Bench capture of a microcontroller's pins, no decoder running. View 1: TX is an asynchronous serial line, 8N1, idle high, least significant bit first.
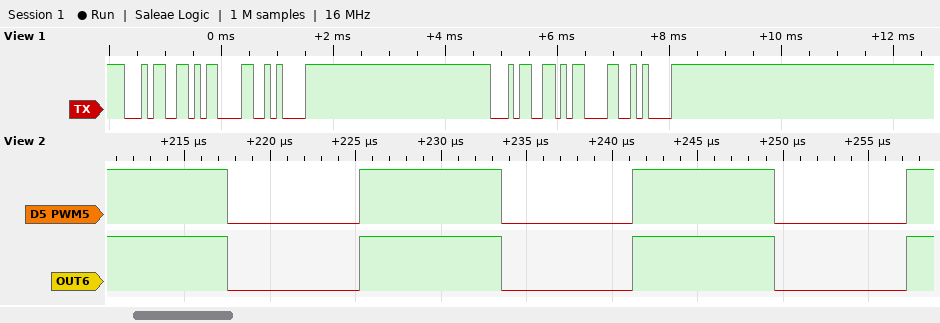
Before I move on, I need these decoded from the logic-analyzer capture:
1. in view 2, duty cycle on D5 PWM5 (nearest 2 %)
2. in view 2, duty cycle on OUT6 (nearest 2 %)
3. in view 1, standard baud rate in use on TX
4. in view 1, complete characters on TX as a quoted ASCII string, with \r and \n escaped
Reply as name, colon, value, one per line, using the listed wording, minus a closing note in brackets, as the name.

in view 2, duty cycle on D5 PWM5: 52 %
in view 2, duty cycle on OUT6: 52 %
in view 1, standard baud rate in use on TX: 9600 baud
in view 1, complete characters on TX as a quoted ASCII string, with \r and \n escaped: "4\r\n4\r\n"
